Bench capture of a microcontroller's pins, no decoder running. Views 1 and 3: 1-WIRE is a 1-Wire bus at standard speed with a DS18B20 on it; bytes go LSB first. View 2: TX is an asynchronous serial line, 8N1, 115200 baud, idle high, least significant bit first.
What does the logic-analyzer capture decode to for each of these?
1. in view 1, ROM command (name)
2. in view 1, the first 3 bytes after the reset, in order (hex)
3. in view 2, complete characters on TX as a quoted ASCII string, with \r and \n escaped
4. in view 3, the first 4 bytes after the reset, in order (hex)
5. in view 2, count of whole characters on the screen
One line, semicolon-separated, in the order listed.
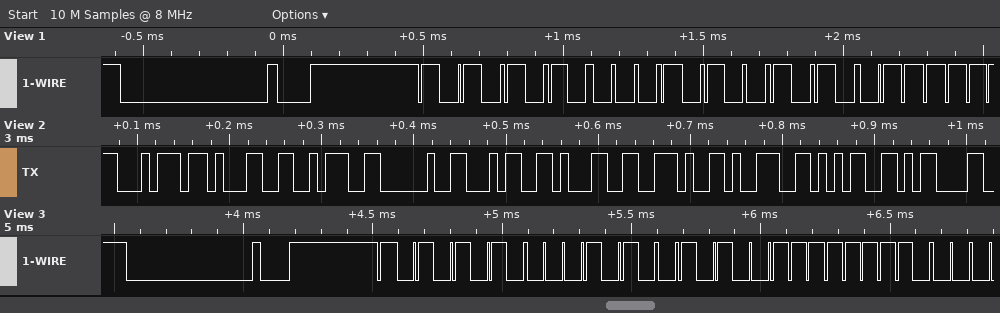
Match ROM; 55 28 E5; "t1: 41.95\r"; 55 28 E5 1F; 10
